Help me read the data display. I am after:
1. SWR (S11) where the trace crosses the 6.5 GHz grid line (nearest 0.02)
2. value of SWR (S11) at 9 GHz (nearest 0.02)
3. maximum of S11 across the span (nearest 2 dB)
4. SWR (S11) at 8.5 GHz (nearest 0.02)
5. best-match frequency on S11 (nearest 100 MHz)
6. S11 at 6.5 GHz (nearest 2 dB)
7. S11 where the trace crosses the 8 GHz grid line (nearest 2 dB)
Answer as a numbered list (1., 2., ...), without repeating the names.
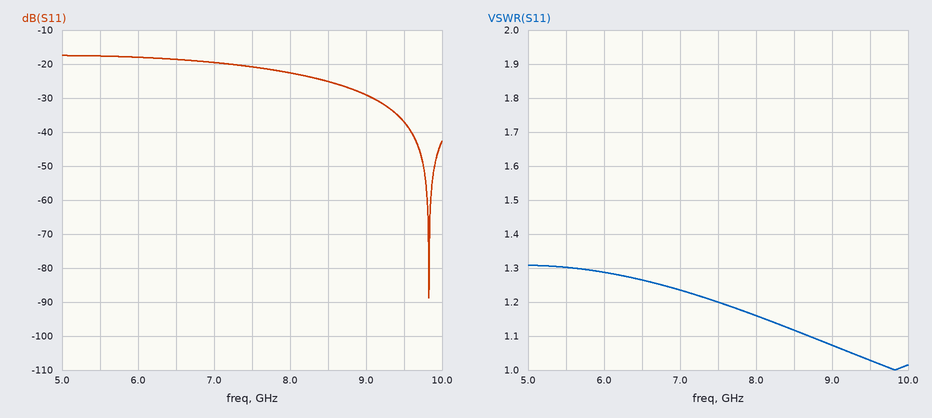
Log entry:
1. 1.26
2. 1.08
3. -18 dB
4. 1.12
5. 9.8 GHz
6. -18 dB
7. -22 dB
